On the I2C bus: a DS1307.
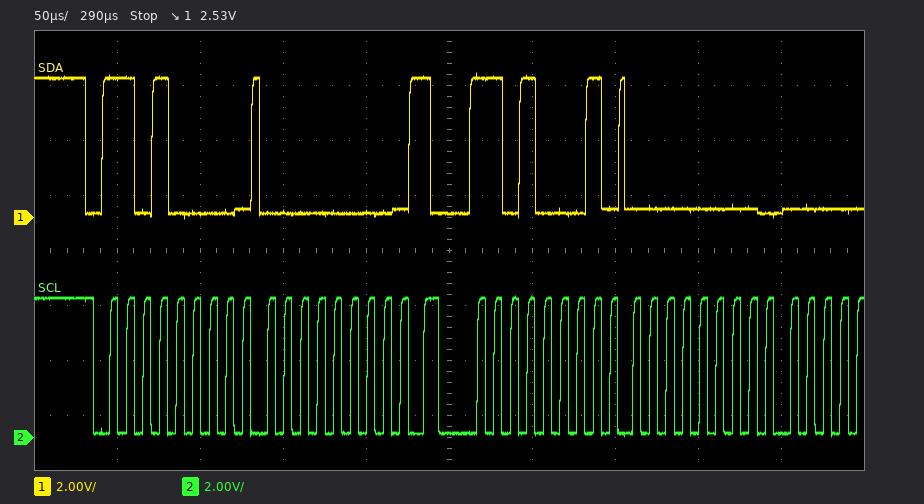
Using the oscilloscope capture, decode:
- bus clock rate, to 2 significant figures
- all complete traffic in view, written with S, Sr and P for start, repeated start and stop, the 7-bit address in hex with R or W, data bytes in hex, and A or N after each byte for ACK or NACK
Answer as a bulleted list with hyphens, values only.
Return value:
- 100 kHz
- S 68W A 00 A Sr 68R A 00 A
